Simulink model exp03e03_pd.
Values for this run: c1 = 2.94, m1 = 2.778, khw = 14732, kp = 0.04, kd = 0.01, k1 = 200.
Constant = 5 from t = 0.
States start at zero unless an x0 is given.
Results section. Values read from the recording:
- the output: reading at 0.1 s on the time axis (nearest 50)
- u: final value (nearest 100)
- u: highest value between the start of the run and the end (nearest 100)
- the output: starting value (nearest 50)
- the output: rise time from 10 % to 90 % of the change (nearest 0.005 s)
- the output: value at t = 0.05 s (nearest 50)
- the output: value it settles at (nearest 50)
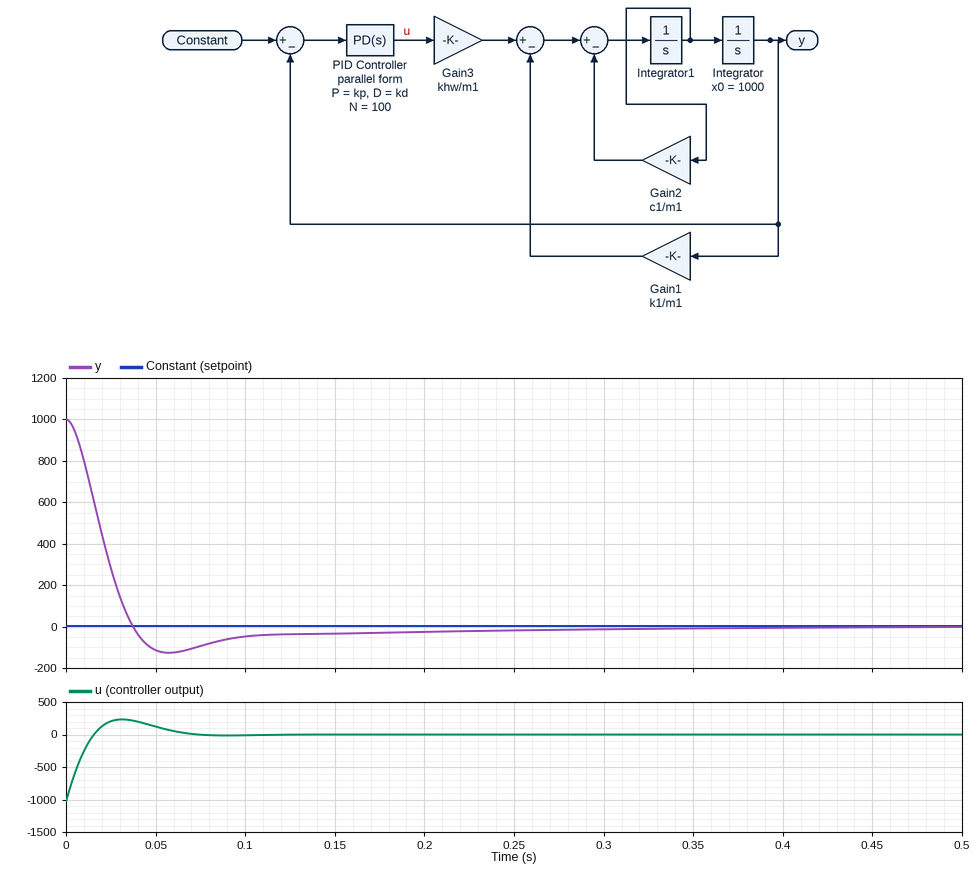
-50
0
200
1000
0.025 s
-100
0
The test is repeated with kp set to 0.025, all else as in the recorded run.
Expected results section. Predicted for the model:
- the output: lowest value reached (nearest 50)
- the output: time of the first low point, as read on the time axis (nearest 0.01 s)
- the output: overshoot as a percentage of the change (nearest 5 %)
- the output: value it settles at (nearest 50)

-100
0.06 s
10 %
0
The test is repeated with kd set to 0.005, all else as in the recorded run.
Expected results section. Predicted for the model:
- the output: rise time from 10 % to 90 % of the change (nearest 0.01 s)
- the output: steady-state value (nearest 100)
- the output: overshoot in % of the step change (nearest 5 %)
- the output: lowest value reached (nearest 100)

0.04 s
0
20 %
-200
